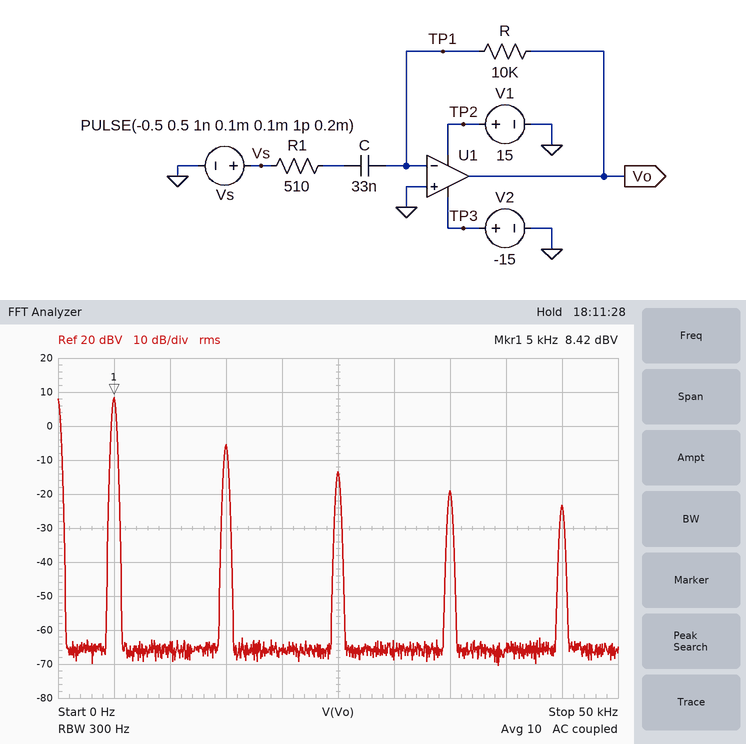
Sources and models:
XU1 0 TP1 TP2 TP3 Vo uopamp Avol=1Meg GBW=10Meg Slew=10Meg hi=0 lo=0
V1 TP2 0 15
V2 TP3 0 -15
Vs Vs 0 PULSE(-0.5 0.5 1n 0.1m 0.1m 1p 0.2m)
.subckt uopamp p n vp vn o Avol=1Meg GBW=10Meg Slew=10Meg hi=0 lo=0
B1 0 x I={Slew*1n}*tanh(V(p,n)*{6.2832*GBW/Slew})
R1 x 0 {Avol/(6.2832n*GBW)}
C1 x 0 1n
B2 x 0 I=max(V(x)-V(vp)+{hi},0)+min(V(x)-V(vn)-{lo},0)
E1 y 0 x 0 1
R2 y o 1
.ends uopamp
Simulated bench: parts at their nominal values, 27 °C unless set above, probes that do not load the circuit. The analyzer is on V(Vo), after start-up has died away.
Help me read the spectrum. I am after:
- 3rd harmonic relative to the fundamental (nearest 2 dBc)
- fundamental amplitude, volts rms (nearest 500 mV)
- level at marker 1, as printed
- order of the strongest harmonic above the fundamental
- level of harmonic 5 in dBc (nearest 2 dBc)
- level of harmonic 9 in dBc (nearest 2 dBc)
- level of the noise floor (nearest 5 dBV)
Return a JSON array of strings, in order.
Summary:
["-14 dBc", "2.5 V", "8.42 dBV", "3", "-22 dBc", "-32 dBc", "-65 dBV"]
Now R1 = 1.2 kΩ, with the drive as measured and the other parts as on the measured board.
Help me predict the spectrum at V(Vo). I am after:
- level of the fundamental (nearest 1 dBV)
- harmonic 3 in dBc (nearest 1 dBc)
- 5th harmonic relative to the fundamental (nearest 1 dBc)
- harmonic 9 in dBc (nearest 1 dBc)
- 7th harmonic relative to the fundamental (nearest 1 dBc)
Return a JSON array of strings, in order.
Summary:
["5 dBV", "-17 dBc", "-26 dBc", "-36 dBc", "-32 dBc"]
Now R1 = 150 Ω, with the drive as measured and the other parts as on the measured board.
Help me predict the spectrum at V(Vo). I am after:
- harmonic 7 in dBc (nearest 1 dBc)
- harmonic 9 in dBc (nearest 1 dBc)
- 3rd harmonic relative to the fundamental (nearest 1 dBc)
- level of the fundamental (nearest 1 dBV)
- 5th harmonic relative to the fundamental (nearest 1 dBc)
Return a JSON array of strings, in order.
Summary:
["-19 dBc", "-23 dBc", "-10 dBc", "9 dBV", "-15 dBc"]
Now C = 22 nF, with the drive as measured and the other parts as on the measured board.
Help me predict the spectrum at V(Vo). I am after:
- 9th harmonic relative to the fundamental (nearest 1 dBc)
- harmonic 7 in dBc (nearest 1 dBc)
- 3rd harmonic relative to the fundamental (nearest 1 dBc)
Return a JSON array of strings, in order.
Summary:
["-29 dBc", "-25 dBc", "-12 dBc"]
